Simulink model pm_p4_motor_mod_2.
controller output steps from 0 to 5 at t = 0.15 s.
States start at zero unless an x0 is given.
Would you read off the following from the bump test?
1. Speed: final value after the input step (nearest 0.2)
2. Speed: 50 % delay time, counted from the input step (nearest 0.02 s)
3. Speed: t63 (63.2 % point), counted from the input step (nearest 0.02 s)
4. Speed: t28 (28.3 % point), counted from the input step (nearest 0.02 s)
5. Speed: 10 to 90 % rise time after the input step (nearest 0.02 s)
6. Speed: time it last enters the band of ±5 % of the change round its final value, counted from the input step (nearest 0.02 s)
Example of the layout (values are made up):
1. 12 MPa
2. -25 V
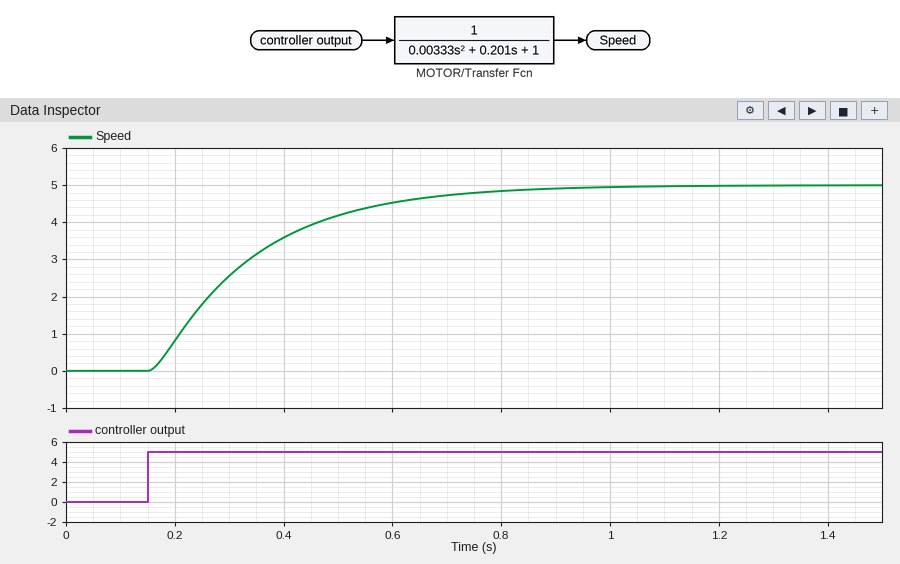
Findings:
1. 5.0
2. 0.14 s
3. 0.20 s
4. 0.08 s
5. 0.40 s
6. 0.56 s
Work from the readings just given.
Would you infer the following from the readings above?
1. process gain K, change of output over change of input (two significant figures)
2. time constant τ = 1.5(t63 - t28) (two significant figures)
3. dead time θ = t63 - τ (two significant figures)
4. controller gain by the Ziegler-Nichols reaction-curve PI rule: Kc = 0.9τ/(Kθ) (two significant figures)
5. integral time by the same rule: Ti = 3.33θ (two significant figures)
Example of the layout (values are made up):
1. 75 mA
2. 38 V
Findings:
1. 1.0
2. 0.18 s
3. 0.020 s
4. 8.1
5. 0.067 s
